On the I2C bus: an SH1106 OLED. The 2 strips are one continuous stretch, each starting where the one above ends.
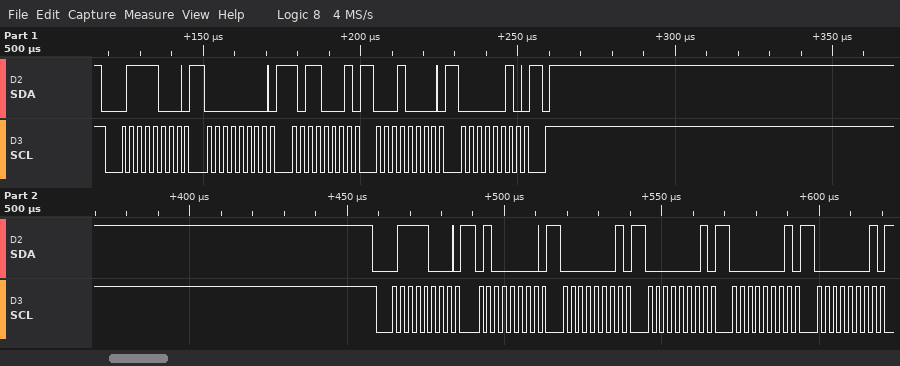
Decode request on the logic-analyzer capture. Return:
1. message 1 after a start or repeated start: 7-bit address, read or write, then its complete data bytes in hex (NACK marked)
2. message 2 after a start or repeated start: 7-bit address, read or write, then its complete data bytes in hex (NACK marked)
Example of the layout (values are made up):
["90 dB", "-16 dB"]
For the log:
["0x3C write: 00 B1 10 02", "0x3C write: 40 01 01 01 01"]
